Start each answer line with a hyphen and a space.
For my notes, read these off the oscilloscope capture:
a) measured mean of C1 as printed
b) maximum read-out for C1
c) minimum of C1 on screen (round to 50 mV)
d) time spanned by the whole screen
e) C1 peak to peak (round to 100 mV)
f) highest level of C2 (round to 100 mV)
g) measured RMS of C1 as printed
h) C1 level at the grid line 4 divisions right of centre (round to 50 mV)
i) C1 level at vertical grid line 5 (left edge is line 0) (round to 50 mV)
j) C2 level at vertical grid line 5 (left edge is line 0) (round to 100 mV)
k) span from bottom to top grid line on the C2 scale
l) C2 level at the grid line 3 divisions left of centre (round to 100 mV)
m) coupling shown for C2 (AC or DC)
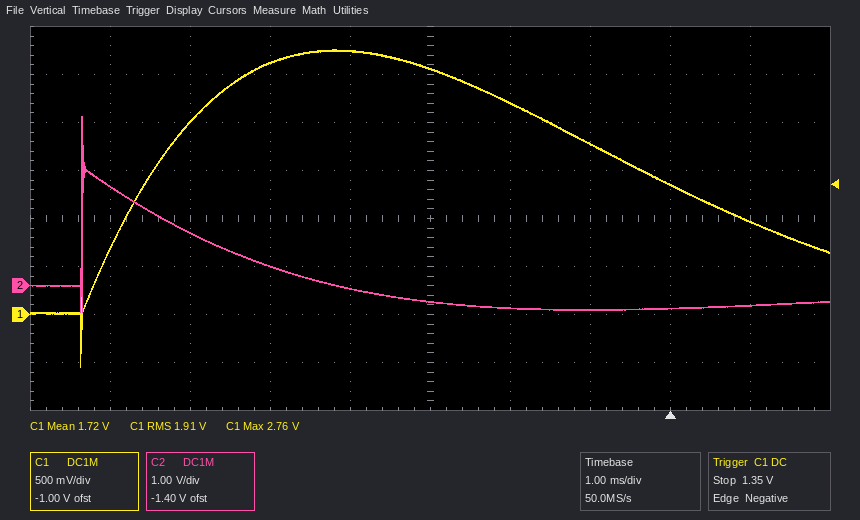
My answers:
- 1.72 V
- 2.76 V
- -550 mV
- 10 ms
- 3.30 V
- 3.5 V
- 1.91 V
- 950 mV
- 2.55 V
- -300 mV
- 8 V
- 1.1 V
- DC
